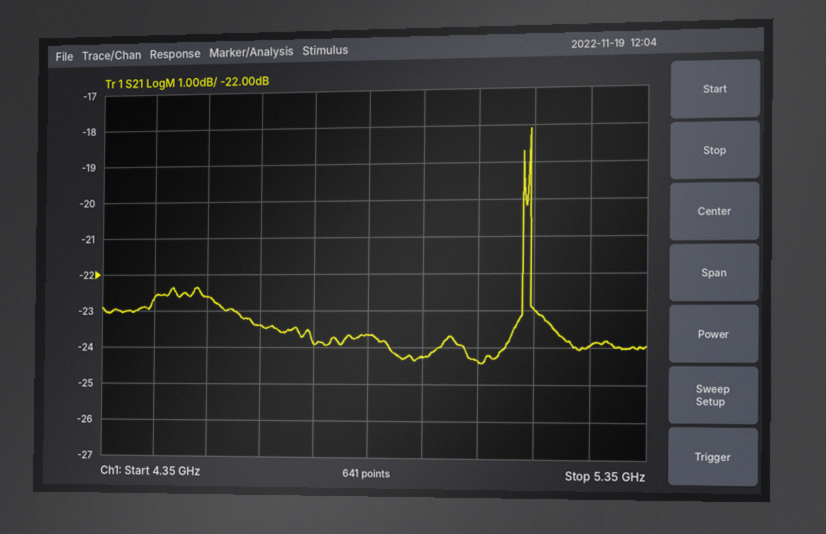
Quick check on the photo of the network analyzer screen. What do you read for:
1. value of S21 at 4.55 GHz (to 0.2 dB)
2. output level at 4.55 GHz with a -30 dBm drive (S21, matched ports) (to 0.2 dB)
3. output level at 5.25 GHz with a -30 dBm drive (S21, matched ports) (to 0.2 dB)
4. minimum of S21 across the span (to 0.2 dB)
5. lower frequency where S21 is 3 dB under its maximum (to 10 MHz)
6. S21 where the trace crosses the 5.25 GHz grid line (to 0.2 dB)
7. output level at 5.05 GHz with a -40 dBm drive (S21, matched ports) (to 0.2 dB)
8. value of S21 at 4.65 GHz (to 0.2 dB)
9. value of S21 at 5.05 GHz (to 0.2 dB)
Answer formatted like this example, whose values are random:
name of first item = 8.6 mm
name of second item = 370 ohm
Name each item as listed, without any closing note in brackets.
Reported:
value of S21 at 4.55 GHz = -22.6 dB
output level at 4.55 GHz with a -30 dBm drive (S21, matched ports) = -52.6 dBm
output level at 5.25 GHz with a -30 dBm drive (S21, matched ports) = -54.0 dBm
minimum of S21 across the span = -24.4 dB
lower frequency where S21 is 3 dB under its maximum = 5.13 GHz
S21 where the trace crosses the 5.25 GHz grid line = -24.0 dB
output level at 5.05 GHz with a -40 dBm drive (S21, matched ports) = -64.4 dBm
value of S21 at 4.65 GHz = -23.4 dB
value of S21 at 5.05 GHz = -24.4 dB
